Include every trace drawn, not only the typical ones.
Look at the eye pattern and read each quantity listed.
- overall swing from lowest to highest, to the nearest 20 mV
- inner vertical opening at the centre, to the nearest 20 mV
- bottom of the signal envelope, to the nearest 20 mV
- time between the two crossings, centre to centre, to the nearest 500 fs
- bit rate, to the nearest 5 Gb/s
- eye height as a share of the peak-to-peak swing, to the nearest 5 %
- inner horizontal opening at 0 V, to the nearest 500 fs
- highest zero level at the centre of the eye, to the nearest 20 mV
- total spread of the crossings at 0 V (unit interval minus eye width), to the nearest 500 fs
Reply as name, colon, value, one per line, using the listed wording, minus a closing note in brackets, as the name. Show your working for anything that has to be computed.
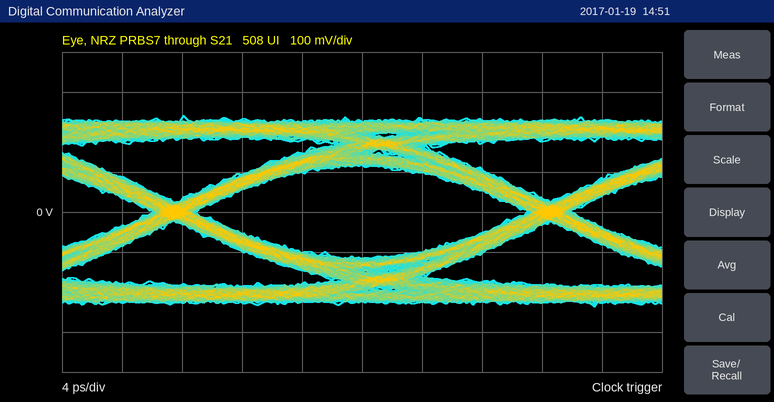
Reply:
overall swing from lowest to highest, to the nearest 20 mV: 480 mV
inner vertical opening at the centre, to the nearest 20 mV: 240 mV
bottom of the signal envelope, to the nearest 20 mV: -240 mV
time between the two crossings, centre to centre, to the nearest 500 fs: 25.0 ps
bit rate, to the nearest 5 Gb/s: 40 Gb/s
eye height as a share of the peak-to-peak swing, to the nearest 5 %: 240 mV / 480 mV ≈ 50 %
inner horizontal opening at 0 V, to the nearest 500 fs: 22.0 ps
highest zero level at the centre of the eye, to the nearest 20 mV: -120 mV
total spread of the crossings at 0 V (unit interval minus eye width), to the nearest 500 fs: 3.0 ps
